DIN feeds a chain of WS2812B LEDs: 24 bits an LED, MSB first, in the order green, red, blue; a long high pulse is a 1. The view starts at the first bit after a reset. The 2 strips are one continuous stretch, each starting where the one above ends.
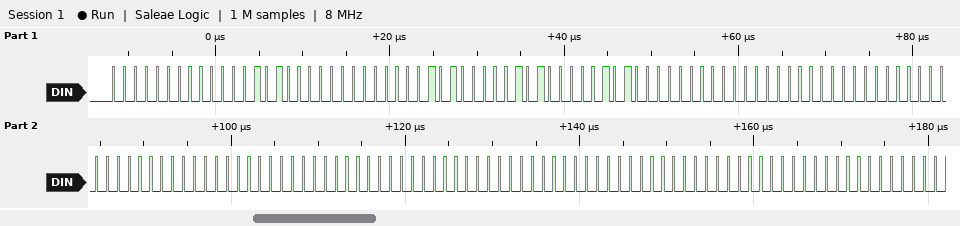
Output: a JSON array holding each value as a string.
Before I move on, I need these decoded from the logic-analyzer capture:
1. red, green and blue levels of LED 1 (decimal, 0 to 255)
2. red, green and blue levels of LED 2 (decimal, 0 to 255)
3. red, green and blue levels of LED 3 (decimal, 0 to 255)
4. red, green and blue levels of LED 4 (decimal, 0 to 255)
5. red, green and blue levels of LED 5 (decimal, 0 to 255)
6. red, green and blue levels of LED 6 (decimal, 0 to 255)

["5, 0, 0", "5, 5, 5", "0, 0, 0", "0, 0, 0", "0, 0, 0", "0, 0, 0"]
